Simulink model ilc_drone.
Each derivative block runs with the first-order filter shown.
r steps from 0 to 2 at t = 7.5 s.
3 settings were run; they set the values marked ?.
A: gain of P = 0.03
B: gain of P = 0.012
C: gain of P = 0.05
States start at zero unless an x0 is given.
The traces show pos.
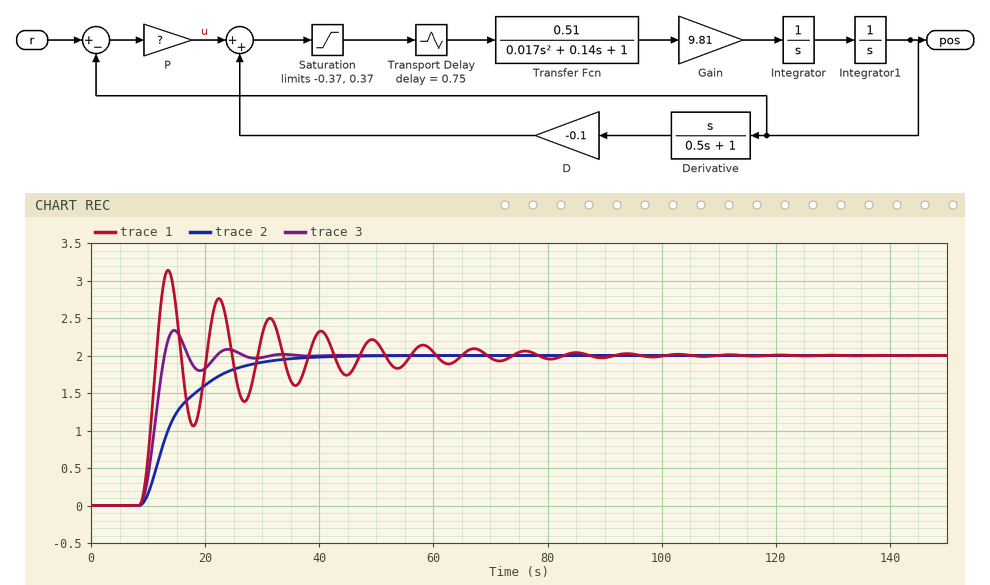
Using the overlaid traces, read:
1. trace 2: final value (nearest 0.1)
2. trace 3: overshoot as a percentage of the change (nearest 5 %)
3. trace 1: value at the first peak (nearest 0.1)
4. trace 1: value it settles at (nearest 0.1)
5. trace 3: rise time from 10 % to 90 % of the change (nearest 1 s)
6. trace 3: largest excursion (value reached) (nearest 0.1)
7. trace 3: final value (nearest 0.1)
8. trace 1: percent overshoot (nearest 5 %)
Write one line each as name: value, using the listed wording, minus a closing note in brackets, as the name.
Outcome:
trace 2: final value: 2.0
trace 3: overshoot as a percentage of the change: 15 %
trace 1: value at the first peak: 3.1
trace 1: value it settles at: 2.0
trace 3: rise time from 10 % to 90 % of the change: 3 s
trace 3: largest excursion (value reached): 2.3
trace 3: final value: 2.0
trace 1: percent overshoot: 55 %
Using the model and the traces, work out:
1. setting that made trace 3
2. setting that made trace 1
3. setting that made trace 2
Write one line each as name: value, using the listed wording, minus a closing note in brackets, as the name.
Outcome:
setting that made trace 3: A
setting that made trace 1: C
setting that made trace 2: B
